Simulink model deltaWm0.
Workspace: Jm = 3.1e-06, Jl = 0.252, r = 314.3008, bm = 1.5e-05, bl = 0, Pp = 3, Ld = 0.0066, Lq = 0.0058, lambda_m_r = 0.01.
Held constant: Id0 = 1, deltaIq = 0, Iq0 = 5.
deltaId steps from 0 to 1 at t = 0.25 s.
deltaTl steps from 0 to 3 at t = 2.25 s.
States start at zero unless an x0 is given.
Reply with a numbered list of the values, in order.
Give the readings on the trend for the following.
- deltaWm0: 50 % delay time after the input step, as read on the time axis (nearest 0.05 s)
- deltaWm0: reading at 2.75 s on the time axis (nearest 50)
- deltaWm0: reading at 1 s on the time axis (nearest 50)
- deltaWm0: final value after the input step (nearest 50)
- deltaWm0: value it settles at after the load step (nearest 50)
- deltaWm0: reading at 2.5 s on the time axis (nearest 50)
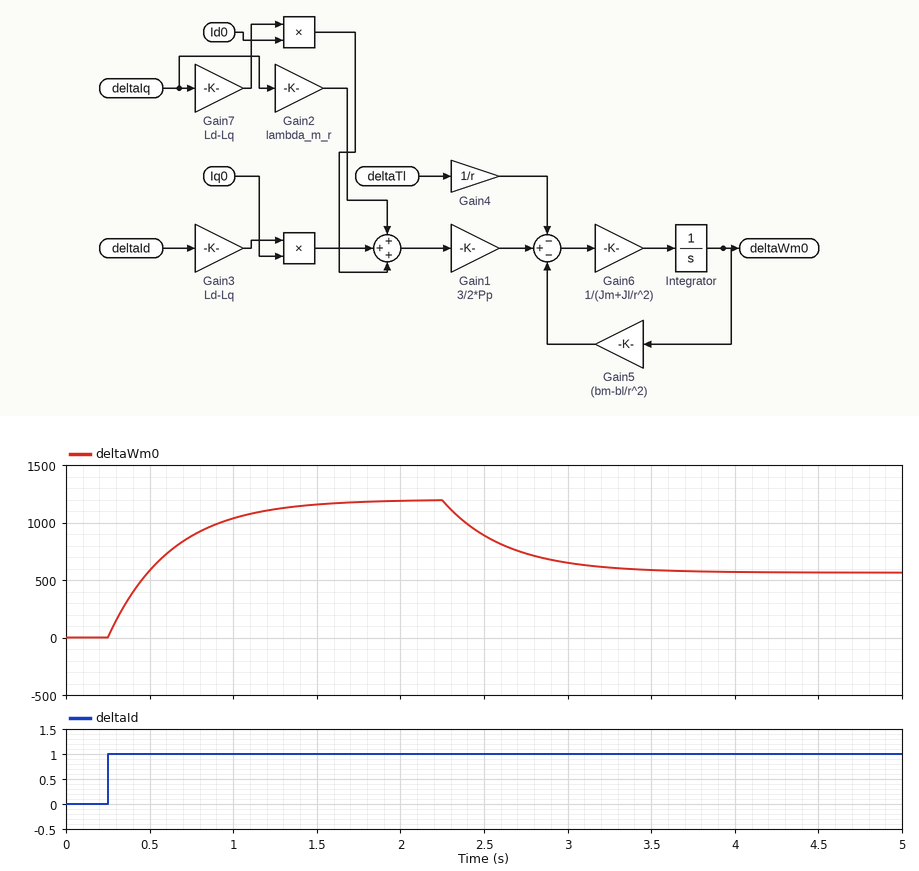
1. 0.50 s
2. 750
3. 1050
4. 1200
5. 550
6. 900
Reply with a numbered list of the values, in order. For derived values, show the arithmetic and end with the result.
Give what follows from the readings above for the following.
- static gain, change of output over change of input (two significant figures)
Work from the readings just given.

1. (1200 - 0) / (1 - 0) = 1200
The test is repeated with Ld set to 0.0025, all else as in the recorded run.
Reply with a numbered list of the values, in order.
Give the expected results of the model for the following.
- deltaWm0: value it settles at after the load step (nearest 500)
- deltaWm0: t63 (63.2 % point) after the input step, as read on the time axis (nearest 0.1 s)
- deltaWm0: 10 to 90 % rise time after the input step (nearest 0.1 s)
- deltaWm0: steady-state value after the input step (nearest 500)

1. -5500
2. 0.6 s
3. 0.8 s
4. -5000
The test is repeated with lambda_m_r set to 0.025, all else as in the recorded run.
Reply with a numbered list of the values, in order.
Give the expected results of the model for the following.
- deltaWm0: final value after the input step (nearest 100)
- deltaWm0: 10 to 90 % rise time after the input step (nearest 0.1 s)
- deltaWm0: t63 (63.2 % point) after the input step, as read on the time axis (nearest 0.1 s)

1. 1200
2. 0.8 s
3. 0.6 s
